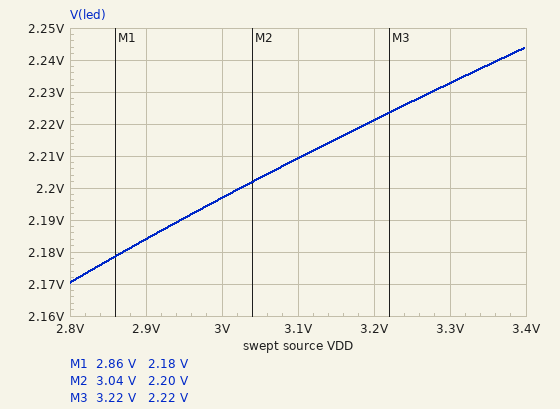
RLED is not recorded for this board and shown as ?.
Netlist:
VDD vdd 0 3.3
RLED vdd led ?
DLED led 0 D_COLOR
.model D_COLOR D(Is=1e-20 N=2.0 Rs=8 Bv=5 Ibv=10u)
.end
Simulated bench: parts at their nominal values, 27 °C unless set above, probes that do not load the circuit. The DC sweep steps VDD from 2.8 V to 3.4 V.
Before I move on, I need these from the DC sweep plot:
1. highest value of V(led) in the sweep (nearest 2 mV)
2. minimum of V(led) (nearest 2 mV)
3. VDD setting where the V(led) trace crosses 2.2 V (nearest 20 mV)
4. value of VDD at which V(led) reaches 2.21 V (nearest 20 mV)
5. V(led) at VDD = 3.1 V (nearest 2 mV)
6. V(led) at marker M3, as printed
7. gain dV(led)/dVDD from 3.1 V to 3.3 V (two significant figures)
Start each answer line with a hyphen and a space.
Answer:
- 2.244 V
- 2.170 V
- 3.02 V
- 3.10 V
- 2.210 V
- 2.22 V
- 0.12 V/V
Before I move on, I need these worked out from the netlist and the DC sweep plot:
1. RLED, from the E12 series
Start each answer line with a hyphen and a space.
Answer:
- 100 Ω
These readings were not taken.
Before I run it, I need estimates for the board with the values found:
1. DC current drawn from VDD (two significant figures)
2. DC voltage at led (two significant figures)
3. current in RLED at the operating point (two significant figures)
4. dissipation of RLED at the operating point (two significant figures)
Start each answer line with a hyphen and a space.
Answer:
- 11 mA
- 2.2 V
- 11 mA
- 11 mW
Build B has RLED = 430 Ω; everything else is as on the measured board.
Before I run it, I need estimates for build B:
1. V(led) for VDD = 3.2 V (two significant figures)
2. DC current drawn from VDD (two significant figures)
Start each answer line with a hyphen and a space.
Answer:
- 2.1 V
- 2.8 mA
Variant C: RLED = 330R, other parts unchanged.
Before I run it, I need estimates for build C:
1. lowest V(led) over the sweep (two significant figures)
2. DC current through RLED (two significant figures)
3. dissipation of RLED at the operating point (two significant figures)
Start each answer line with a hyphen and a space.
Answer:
- 2.1 V
- 3.6 mA
- 4.2 mW
